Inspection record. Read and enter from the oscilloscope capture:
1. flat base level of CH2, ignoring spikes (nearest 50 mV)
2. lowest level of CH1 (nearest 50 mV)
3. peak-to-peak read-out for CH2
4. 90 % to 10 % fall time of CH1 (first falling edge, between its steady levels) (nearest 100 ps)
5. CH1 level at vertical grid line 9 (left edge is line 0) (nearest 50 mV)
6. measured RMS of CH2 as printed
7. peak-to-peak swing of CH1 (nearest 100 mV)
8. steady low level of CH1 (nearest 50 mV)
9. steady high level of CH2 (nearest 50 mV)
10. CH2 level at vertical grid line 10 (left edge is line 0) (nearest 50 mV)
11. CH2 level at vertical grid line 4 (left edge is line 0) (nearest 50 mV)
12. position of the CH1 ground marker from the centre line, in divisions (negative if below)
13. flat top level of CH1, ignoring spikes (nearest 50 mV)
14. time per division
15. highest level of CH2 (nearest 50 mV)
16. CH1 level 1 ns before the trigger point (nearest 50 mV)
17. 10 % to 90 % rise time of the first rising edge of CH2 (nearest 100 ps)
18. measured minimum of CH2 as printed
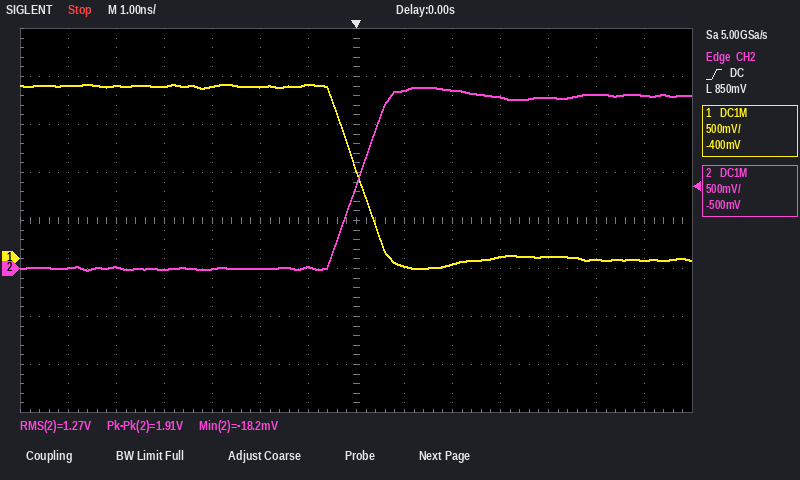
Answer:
0 mV
-100 mV
1.91 V
1.0 ns
-50 mV
1.27 V
1.90 V
0 mV
1.80 V
1.80 V
0 mV
-0.8 div
1.80 V
1 ns
1.90 V
1.80 V
1.0 ns
-18.2 mV
